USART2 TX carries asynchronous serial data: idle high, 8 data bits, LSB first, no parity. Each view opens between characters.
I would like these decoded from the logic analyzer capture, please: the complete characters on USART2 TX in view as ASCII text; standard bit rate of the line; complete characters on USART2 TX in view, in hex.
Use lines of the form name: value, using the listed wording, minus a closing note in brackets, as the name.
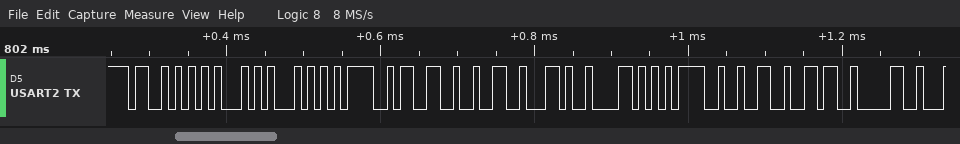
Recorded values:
the complete characters on USART2 TX in view as ASCII text: "SEQ=32,X=260"
standard bit rate of the line: 115200 baud
complete characters on USART2 TX in view, in hex: 53, 45, 51, 3D, 33, 32, 2C, 58, 3D, 32, 36, 30
